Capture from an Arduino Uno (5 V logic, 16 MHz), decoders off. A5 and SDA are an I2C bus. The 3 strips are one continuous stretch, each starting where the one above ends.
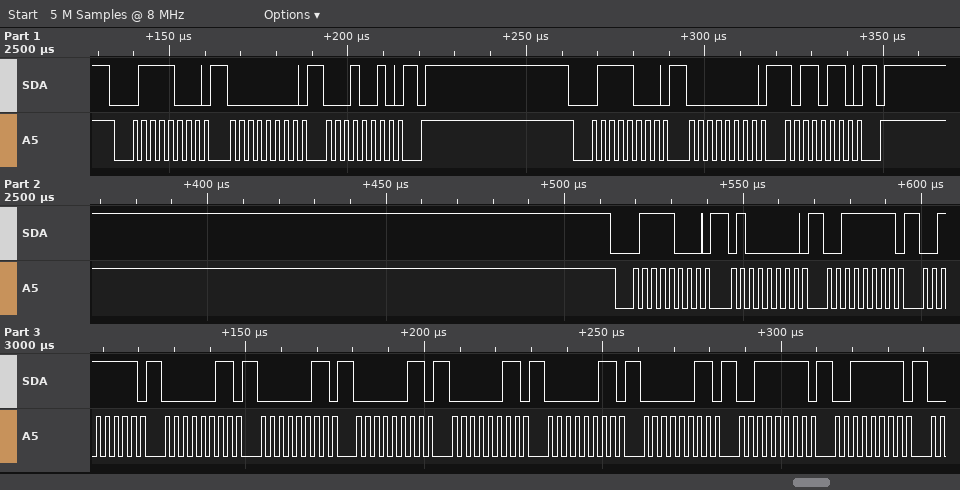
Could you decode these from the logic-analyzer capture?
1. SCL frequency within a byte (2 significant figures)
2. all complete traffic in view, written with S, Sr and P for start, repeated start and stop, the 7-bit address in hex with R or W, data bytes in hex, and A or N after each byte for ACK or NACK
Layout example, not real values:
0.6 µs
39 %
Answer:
400 kHz
S 3CW A 00 A 12 A P S 3CW A 00 A B6 A P S 3CW A 40 A 3F A 3F A 03 A 03 A 03 A 03 A 03 A 03 A 3F A 3F A
